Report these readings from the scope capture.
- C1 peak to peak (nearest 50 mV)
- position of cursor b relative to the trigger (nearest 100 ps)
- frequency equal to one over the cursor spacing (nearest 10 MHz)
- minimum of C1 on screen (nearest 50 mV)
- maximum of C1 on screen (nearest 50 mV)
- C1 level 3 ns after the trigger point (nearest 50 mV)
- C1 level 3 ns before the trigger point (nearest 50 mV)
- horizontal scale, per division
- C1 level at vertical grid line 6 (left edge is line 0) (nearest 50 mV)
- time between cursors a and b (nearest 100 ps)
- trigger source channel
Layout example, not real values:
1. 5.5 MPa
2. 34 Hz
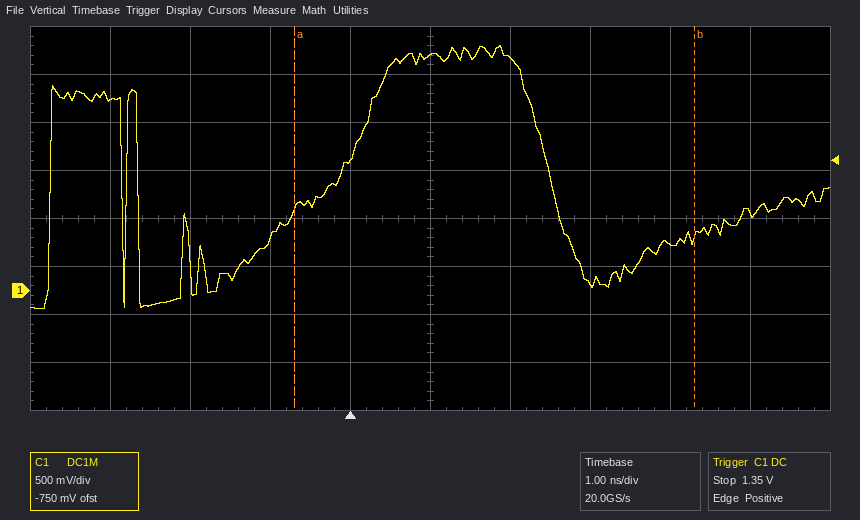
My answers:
1. 2.75 V
2. +4.3 ns
3. 200 MHz
4. -200 mV
5. 2.55 V
6. 50 mV
7. 2.00 V
8. 1 ns
9. 2.40 V
10. 5.0 ns
11. C1
